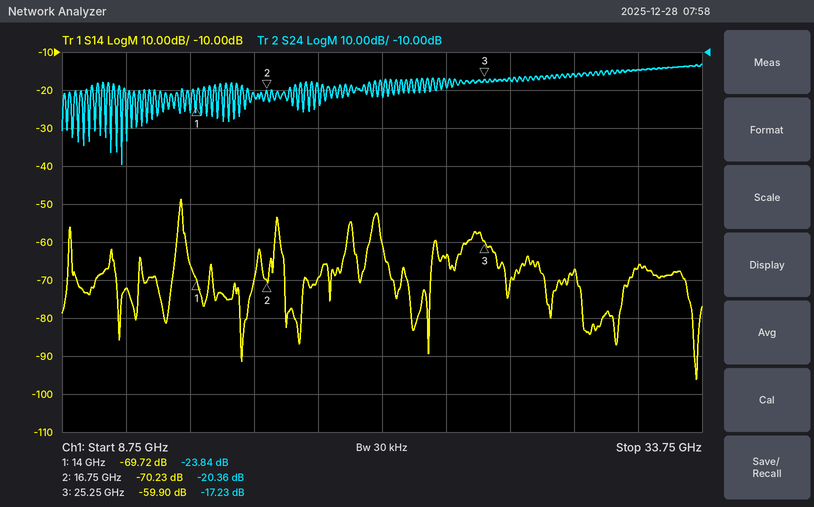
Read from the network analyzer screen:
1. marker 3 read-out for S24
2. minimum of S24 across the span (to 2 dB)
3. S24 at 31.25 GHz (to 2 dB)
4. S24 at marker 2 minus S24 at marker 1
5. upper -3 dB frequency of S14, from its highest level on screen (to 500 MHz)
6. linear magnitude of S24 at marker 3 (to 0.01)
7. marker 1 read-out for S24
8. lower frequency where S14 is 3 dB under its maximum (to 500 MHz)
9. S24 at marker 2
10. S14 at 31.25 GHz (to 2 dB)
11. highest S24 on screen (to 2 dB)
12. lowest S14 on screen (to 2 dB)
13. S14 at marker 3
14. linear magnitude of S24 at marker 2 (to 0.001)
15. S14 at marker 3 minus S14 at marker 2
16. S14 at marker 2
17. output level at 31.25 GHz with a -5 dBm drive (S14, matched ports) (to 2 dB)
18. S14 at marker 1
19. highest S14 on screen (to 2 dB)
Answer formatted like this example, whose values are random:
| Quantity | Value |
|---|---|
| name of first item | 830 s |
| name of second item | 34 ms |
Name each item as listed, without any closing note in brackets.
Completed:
| Quantity | Value |
|---|---|
| marker 3 read-out for S24 | -17.23 dB |
| minimum of S24 across the span | -40 dB |
| S24 at 31.25 GHz | -14 dB |
| S24 at marker 2 minus S24 at marker 1 | 3.48 dB |
| upper -3 dB frequency of S14, from its highest level on screen | 13.5 GHz |
| linear magnitude of S24 at marker 3 | 0.14 |
| marker 1 read-out for S24 | -23.84 dB |
| lower frequency where S14 is 3 dB under its maximum | 13.5 GHz |
| S24 at marker 2 | -20.36 dB |
| S14 at 31.25 GHz | -66 dB |
| highest S24 on screen | -14 dB |
| lowest S14 on screen | -96 dB |
| S14 at marker 3 | -59.90 dB |
| linear magnitude of S24 at marker 2 | 0.096 |
| S14 at marker 3 minus S14 at marker 2 | 10.33 dB |
| S14 at marker 2 | -70.23 dB |
| output level at 31.25 GHz with a -5 dBm drive (S14, matched ports) | -72 dBm |
| S14 at marker 1 | -69.72 dB |
| highest S14 on screen | -48 dB |
